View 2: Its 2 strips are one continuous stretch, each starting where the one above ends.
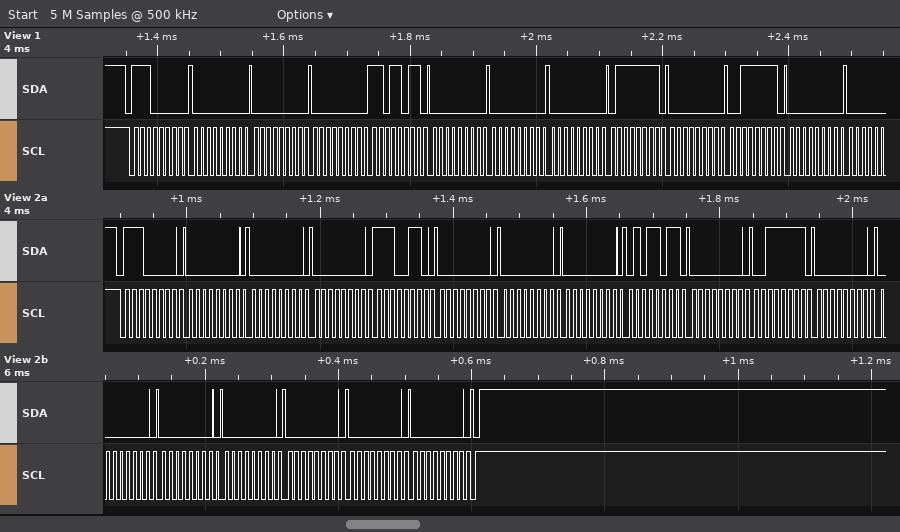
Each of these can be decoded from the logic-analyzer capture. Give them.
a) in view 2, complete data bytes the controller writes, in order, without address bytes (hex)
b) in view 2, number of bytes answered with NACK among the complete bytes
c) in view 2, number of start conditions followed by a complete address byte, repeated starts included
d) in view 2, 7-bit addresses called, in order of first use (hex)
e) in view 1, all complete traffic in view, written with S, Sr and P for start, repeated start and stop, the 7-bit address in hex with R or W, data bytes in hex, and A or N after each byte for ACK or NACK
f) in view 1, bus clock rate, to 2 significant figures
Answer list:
00 00 00 E6 00 00 00 5B 00 3F 00 00 00 00 00 00 00
0
1
0x70
S 70W A 00 A 00 A 00 A DB A 00 A 00 A 00 A 7F A 00 A 3F A 00 A
100 kHz
